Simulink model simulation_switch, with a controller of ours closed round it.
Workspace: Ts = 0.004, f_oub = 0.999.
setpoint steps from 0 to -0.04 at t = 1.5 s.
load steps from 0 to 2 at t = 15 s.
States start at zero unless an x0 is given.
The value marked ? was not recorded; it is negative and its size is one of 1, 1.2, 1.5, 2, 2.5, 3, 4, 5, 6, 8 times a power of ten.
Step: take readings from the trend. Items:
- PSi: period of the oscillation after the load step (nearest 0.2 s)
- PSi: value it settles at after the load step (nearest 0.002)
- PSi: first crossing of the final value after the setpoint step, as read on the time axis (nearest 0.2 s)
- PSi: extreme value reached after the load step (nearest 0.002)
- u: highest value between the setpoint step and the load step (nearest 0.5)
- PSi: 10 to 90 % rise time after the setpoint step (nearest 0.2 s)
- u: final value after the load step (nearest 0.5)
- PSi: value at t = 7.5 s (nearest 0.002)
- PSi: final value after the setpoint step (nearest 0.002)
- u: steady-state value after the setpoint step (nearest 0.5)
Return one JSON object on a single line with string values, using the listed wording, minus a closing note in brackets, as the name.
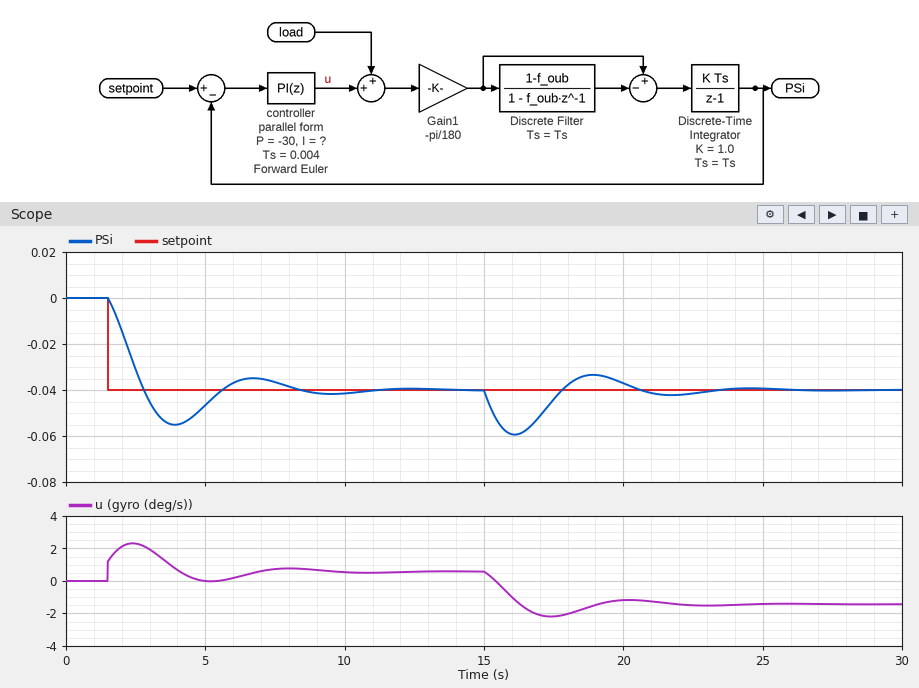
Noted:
{"PSi: period of the oscillation after the load step": "5.6 s", "PSi: value it settles at after the load step": "-0.040", "PSi: first crossing of the final value after the setpoint step, as read on the time axis": "2.8 s", "PSi: extreme value reached after the load step": "-0.060", "u: highest value between the setpoint step and the load step": "2.5", "PSi: 10 to 90 % rise time after the setpoint step": "1.0 s", "u: final value after the load step": "-1.5", "PSi: value at t = 7.5 s": "-0.036", "PSi: final value after the setpoint step": "-0.040", "u: steady-state value after the setpoint step": "0.5"}
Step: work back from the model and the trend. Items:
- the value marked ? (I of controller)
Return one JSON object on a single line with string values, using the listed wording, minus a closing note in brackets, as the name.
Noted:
{"the value marked ?": "-80"}
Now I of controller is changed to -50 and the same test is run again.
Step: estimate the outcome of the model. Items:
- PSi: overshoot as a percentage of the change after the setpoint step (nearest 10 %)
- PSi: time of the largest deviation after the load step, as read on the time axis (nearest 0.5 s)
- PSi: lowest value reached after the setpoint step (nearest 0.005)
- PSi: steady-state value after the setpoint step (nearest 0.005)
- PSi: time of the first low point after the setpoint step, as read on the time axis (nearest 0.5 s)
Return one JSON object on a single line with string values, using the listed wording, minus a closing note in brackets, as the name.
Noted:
{"PSi: overshoot as a percentage of the change after the setpoint step": "30 %", "PSi: time of the largest deviation after the load step, as read on the time axis": "16.5 s", "PSi: lowest value reached after the setpoint step": "-0.050", "PSi: steady-state value after the setpoint step": "-0.040", "PSi: time of the first low point after the setpoint step, as read on the time axis": "4.5 s"}
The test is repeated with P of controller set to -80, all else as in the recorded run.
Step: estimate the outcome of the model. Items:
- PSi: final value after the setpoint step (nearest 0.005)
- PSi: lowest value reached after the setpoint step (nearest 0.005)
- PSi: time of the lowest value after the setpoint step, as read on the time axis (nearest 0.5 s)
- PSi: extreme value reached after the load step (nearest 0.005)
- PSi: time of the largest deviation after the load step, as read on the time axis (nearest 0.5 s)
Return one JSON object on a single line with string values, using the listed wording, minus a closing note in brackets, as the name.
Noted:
{"PSi: final value after the setpoint step": "-0.040", "PSi: lowest value reached after the setpoint step": "-0.045", "PSi: time of the lowest value after the setpoint step, as read on the time axis": "3.5 s", "PSi: extreme value reached after the load step": "-0.055", "PSi: time of the largest deviation after the load step, as read on the time axis": "16.0 s"}
